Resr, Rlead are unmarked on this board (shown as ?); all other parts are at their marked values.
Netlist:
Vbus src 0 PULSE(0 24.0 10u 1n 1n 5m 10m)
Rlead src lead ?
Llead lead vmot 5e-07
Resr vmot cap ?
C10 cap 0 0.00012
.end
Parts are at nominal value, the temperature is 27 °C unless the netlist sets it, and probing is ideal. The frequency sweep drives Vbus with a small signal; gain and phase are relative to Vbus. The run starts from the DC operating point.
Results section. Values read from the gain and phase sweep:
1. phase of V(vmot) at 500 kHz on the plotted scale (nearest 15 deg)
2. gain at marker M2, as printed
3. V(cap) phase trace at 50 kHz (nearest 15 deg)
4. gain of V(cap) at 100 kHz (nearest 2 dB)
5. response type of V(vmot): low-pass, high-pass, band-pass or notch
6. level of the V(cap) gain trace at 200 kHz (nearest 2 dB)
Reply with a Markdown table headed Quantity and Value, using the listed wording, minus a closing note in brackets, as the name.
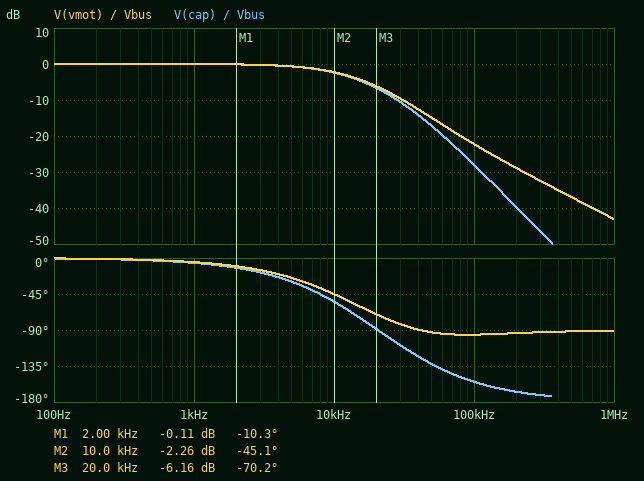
| Quantity | Value |
|---|---|
| phase of V(vmot) at 500 kHz on the plotted scale | -90 deg |
| gain at marker M2, as printed | -2.26 dB |
| V(cap) phase trace at 50 kHz | -135 deg |
| gain of V(cap) at 100 kHz | -28 dB |
| response type of V(vmot): low-pass, high-pass, band-pass or notch | low-pass |
| level of the V(cap) gain trace at 200 kHz | -40 dB |
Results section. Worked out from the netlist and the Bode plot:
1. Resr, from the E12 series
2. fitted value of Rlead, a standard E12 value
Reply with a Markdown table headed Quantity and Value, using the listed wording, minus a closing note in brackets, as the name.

| Quantity | Value |
|---|---|
| Resr, from the E12 series | 0.022 Ω |
| fitted value of Rlead, a standard E12 value | 0.12 Ω |
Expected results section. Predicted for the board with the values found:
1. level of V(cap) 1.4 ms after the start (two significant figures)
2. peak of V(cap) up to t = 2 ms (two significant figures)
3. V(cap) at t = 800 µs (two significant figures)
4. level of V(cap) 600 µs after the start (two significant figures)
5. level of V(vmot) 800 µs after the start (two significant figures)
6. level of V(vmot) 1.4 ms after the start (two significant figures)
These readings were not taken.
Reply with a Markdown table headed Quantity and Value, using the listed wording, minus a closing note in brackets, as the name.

| Quantity | Value |
|---|---|
| level of V(cap) 1.4 ms after the start | 24 V |
| peak of V(cap) up to t = 2 ms | 24 V |
| V(cap) at t = 800 µs | 24 V |
| level of V(cap) 600 µs after the start | 24 V |
| level of V(vmot) 800 µs after the start | 24 V |
| level of V(vmot) 1.4 ms after the start | 24 V |
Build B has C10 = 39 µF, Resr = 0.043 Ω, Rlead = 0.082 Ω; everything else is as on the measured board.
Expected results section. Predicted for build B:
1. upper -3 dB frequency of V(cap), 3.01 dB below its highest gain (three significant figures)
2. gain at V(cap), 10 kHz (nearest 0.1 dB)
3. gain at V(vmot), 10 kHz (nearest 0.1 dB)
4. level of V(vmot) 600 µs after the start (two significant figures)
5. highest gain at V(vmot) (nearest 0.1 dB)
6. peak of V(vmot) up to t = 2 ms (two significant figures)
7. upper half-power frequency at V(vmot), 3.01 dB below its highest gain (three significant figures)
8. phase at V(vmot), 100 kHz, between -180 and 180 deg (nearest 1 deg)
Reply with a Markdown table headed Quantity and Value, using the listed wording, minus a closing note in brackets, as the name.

| Quantity | Value |
|---|---|
| upper -3 dB frequency of V(cap), 3.01 dB below its highest gain | 41.3 kHz |
| gain at V(cap), 10 kHz | 0.2 dB |
| gain at V(vmot), 10 kHz | 0.3 dB |
| level of V(vmot) 600 µs after the start | 24 V |
| highest gain at V(vmot) | 1.0 dB |
| peak of V(vmot) up to t = 2 ms | 27 V |
| upper half-power frequency at V(vmot), 3.01 dB below its highest gain | 43.1 kHz |
| phase at V(vmot), 100 kHz, between -180 and 180 deg | -109 deg |
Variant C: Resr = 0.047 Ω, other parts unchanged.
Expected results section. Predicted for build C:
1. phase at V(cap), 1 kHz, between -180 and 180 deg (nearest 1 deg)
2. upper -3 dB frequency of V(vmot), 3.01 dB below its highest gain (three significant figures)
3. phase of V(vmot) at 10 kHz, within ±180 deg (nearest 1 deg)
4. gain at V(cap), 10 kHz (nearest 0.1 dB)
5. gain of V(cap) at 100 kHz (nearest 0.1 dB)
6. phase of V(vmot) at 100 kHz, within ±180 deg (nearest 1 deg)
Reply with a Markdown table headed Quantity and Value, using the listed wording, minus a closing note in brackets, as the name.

| Quantity | Value |
|---|---|
| phase at V(cap), 1 kHz, between -180 and 180 deg | -7 deg |
| upper -3 dB frequency of V(vmot), 3.01 dB below its highest gain | 10.4 kHz |
| phase of V(vmot) at 10 kHz, within ±180 deg | -39 deg |
| gain at V(cap), 10 kHz | -3.4 dB |
| gain of V(cap) at 100 kHz | -28.3 dB |
| phase of V(vmot) at 100 kHz, within ±180 deg | -77 deg |
